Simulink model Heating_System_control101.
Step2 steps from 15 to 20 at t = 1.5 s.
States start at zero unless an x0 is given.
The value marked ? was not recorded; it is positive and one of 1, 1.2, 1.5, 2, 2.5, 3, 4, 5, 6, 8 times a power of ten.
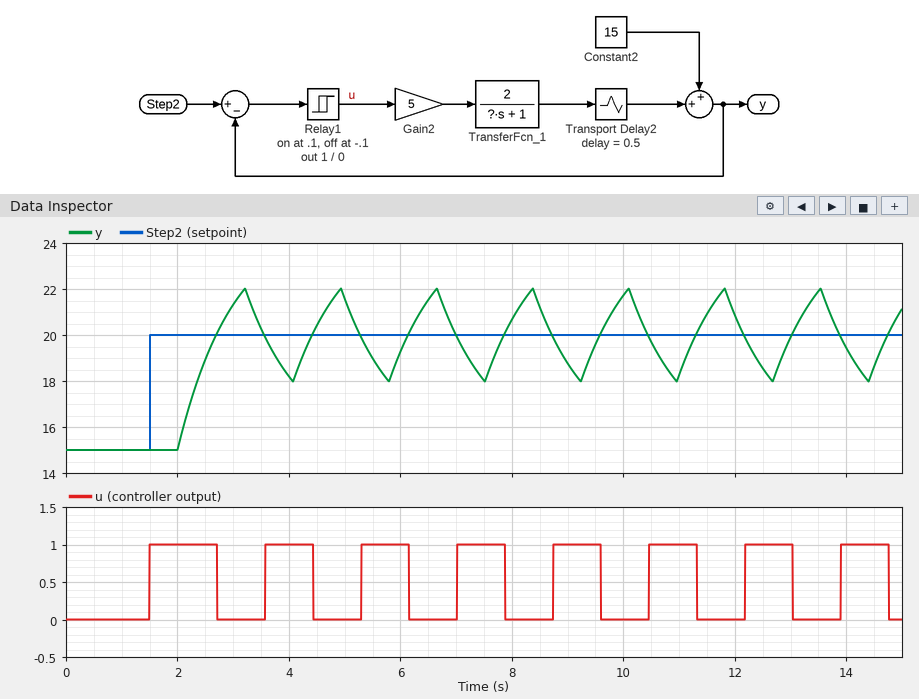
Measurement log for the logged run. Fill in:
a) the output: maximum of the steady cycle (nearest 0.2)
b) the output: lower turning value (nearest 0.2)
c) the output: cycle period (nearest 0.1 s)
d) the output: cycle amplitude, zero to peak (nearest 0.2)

22.0
18.0
1.7 s
2.0
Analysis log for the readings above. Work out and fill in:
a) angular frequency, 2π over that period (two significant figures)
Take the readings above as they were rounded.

3.7 rad/s
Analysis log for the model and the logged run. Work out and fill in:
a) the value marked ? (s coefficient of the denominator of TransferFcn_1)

1
